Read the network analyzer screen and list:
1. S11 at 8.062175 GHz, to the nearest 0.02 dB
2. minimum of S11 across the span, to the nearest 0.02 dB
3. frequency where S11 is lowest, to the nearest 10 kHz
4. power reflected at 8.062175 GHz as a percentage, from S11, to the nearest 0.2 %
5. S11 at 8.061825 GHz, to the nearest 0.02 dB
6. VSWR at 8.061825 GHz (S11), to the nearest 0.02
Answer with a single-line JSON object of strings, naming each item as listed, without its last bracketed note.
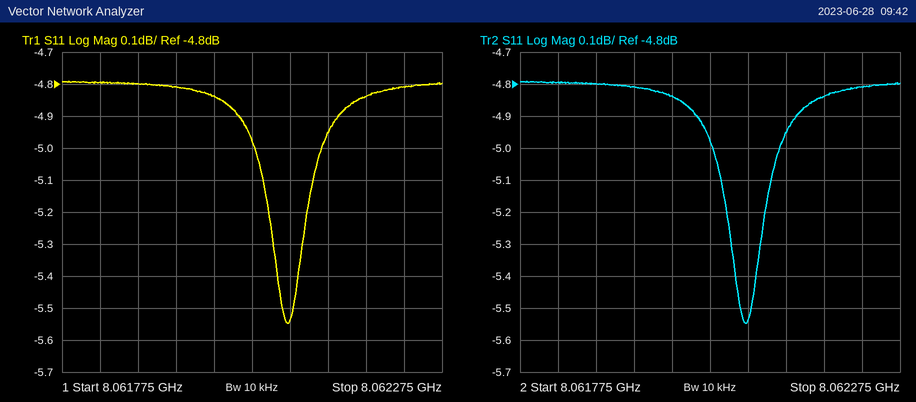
{"S11 at 8.062175 GHz, to the nearest 0.02 dB": "-4.84 dB", "minimum of S11 across the span, to the nearest 0.02 dB": "-5.54 dB", "frequency where S11 is lowest, to the nearest 10 kHz": "8.06207 GHz", "power reflected at 8.062175 GHz as a percentage, from S11, to the nearest 0.2 %": "32.8 %", "S11 at 8.061825 GHz, to the nearest 0.02 dB": "-4.80 dB", "VSWR at 8.061825 GHz (S11), to the nearest 0.02": "3.72"}
